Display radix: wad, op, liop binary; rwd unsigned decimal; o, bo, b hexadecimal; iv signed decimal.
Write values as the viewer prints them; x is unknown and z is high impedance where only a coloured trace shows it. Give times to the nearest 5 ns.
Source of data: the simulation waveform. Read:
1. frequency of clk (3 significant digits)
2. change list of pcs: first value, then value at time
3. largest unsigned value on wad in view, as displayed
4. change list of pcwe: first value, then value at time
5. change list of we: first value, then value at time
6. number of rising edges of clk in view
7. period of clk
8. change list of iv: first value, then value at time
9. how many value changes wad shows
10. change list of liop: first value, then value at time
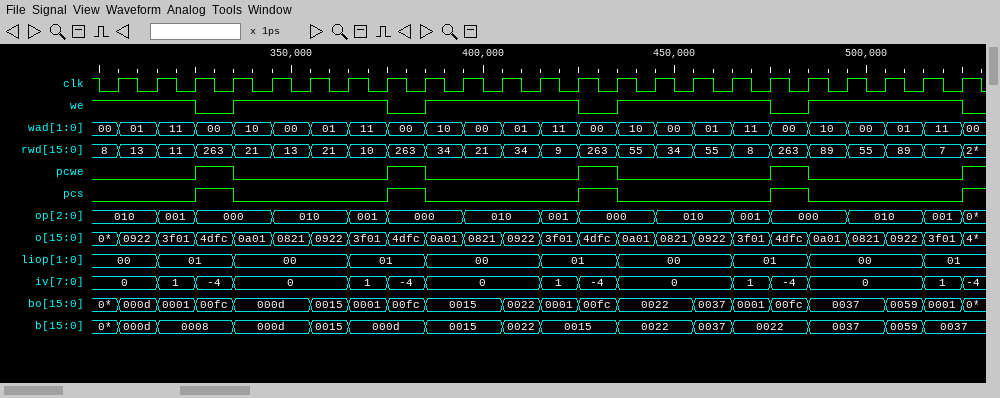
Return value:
100 MHz
0, 1 at 325 ns, 0 at 335 ns, 1 at 375 ns, 0 at 385 ns, 1 at 425 ns, 0 at 435 ns, 1 at 475 ns, 0 at 485 ns, 1 at 525 ns
11
0, 1 at 325 ns, 0 at 335 ns, 1 at 375 ns, 0 at 385 ns, 1 at 425 ns, 0 at 435 ns, 1 at 475 ns, 0 at 485 ns, 1 at 525 ns
1, 0 at 325 ns, 1 at 335 ns, 0 at 375 ns, 1 at 385 ns, 0 at 425 ns, 1 at 435 ns, 0 at 475 ns, 1 at 485 ns, 0 at 525 ns
23
10 ns
0, 1 at 315 ns, -4 at 325 ns, 0 at 335 ns, 1 at 365 ns, -4 at 375 ns, 0 at 385 ns, 1 at 415 ns, -4 at 425 ns, 0 at 435 ns, 1 at 465 ns, -4 at 475 ns, 0 at 485 ns, 1 at 515 ns, -4 at 525 ns
23
00, 01 at 315 ns, 00 at 335 ns, 01 at 365 ns, 00 at 385 ns, 01 at 415 ns, 00 at 435 ns, 01 at 465 ns, 00 at 485 ns, 01 at 515 ns
